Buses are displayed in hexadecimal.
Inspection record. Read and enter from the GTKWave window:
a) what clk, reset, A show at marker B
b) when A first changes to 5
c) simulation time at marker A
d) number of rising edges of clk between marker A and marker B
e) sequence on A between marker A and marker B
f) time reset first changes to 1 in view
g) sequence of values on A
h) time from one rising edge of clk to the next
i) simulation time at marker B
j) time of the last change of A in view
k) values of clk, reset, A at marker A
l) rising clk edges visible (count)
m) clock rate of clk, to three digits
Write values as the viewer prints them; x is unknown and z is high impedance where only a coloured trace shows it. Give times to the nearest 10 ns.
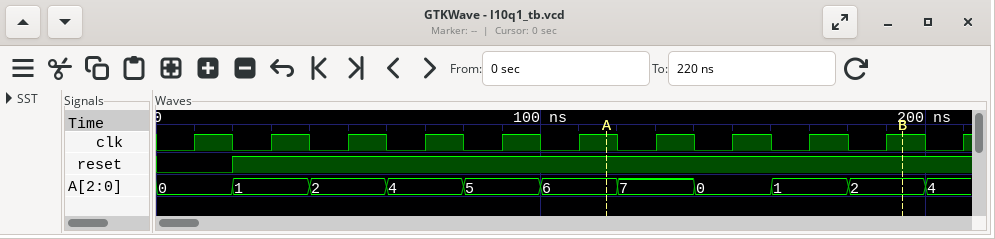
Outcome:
clk=1, reset=1, A=2
80 ns
120 ns
4
6, 7, 0, 1, 2
20 ns
0, 1, 2, 4, 5, 6, 7, 0, 1, 2, 4
20 ns
190 ns
200 ns
clk=1, reset=1, A=6
11
50.0 MHz
